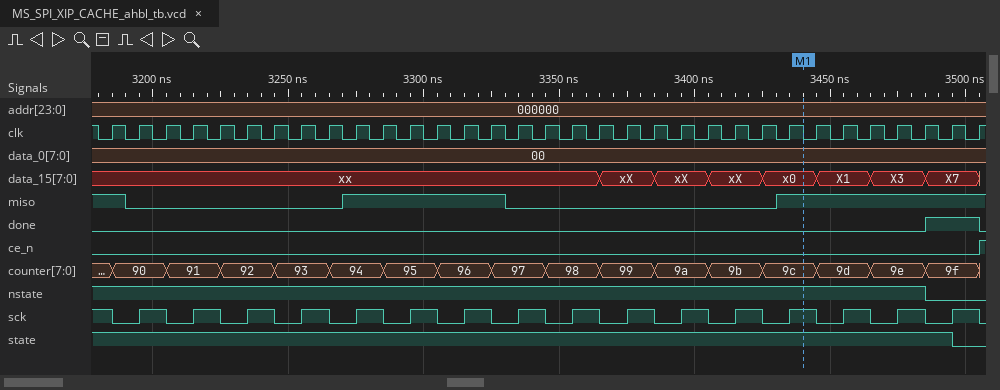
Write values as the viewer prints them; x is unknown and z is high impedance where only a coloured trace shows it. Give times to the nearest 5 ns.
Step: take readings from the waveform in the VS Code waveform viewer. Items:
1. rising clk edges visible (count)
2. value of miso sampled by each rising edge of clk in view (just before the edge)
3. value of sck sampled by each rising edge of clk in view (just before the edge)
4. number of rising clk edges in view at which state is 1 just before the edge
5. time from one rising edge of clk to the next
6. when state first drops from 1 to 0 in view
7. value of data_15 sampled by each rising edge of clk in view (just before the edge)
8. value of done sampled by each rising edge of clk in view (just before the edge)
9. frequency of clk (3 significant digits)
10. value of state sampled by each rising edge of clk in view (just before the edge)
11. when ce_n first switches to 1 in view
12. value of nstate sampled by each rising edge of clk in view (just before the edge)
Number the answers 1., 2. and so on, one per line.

1. 33
2. 1 0 0 0 0 0 0 0 0 1 1 1 1 1 1 0 0 0 0 0 0 0 0 0 0 1 1 1 1 1 1 1 1
3. 1 0 1 0 1 0 1 0 1 0 1 0 1 0 1 0 1 0 1 0 1 0 1 0 1 0 1 0 1 0 1 0 1
4. 32
5. 10 ns
6. 3495 ns
7. xx, xx, xx, xx, xx, xx, xx, xx, xx, xx, xx, xx, xx, xx, xx, xx, xx, xx, xx, xX, xX, xX, xX, xX, xX, x0, x0, X1, X1, X3, X3, X7, X7
8. 0 0 0 0 0 0 0 0 0 0 0 0 0 0 0 0 0 0 0 0 0 0 0 0 0 0 0 0 0 0 0 1 1
9. 100 MHz
10. 1 1 1 1 1 1 1 1 1 1 1 1 1 1 1 1 1 1 1 1 1 1 1 1 1 1 1 1 1 1 1 1 0
11. 3505 ns
12. 1 1 1 1 1 1 1 1 1 1 1 1 1 1 1 1 1 1 1 1 1 1 1 1 1 1 1 1 1 1 1 0 0
